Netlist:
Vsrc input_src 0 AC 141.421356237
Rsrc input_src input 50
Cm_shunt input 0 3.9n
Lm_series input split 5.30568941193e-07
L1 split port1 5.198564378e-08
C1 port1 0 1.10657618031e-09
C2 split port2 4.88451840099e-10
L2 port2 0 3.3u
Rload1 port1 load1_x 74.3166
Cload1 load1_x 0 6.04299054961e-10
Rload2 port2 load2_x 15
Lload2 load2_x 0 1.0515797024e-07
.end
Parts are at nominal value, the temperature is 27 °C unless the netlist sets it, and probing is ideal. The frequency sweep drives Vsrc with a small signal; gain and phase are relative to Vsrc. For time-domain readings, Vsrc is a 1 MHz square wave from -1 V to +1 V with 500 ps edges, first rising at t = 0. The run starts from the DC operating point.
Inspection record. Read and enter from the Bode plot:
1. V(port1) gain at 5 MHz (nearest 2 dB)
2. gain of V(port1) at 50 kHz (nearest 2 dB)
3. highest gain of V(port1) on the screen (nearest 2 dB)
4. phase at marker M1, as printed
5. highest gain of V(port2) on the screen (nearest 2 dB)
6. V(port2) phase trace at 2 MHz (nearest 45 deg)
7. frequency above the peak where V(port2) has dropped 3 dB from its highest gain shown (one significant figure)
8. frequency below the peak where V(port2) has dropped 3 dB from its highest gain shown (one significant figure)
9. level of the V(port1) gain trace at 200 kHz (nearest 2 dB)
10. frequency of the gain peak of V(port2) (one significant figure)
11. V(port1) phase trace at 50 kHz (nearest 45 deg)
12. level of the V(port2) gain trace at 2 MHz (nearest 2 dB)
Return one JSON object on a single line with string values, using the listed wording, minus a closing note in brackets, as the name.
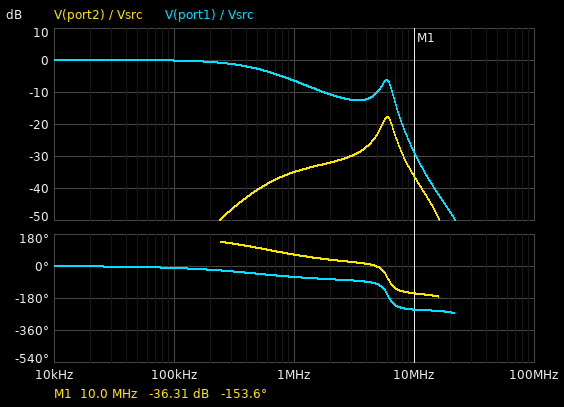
{"V(port1) gain at 5 MHz": "-10 dB", "gain of V(port1) at 50 kHz": "0 dB", "highest gain of V(port1) on the screen": "0 dB", "phase at marker M1, as printed": "-153.6 deg", "highest gain of V(port2) on the screen": "-18 dB", "V(port2) phase trace at 2 MHz": "45 deg", "frequency above the peak where V(port2) has dropped 3 dB from its highest gain shown": "7 MHz", "frequency below the peak where V(port2) has dropped 3 dB from its highest gain shown": "5 MHz", "level of the V(port1) gain trace at 200 kHz": "0 dB", "frequency of the gain peak of V(port2)": "6 MHz", "V(port1) phase trace at 50 kHz": "0 deg", "level of the V(port2) gain trace at 2 MHz": "-32 dB"}
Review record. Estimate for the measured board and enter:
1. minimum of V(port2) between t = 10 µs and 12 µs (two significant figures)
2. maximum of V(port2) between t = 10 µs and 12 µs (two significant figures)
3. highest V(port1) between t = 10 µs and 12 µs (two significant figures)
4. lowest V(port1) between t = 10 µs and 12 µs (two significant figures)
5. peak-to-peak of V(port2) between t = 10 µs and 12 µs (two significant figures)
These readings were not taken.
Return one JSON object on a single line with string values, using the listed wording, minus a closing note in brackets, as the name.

{"minimum of V(port2) between t = 10 µs and 12 µs": "-65 mV", "maximum of V(port2) between t = 10 µs and 12 µs": "65 mV", "highest V(port1) between t = 10 µs and 12 µs": "670 mV", "lowest V(port1) between t = 10 µs and 12 µs": "-670 mV", "peak-to-peak of V(port2) between t = 10 µs and 12 µs": "130 mV"}
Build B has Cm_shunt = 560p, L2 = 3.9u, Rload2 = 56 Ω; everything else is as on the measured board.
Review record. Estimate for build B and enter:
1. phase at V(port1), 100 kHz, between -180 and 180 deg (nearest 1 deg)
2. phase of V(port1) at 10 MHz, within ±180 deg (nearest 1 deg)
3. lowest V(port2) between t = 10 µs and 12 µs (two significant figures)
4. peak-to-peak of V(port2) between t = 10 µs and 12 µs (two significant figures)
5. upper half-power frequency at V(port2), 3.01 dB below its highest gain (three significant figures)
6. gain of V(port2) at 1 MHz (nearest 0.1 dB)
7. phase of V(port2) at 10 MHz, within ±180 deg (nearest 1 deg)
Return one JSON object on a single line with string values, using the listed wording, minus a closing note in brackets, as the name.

{"phase at V(port1), 100 kHz, between -180 and 180 deg": "-5 deg", "phase of V(port1) at 10 MHz, within ±180 deg": "-144 deg", "lowest V(port2) between t = 10 µs and 12 µs": "-330 mV", "peak-to-peak of V(port2) between t = 10 µs and 12 µs": "660 mV", "upper half-power frequency at V(port2), 3.01 dB below its highest gain": "11.4 MHz", "gain of V(port2) at 1 MHz": "-25.2 dB", "phase of V(port2) at 10 MHz, within ±180 deg": "-106 deg"}
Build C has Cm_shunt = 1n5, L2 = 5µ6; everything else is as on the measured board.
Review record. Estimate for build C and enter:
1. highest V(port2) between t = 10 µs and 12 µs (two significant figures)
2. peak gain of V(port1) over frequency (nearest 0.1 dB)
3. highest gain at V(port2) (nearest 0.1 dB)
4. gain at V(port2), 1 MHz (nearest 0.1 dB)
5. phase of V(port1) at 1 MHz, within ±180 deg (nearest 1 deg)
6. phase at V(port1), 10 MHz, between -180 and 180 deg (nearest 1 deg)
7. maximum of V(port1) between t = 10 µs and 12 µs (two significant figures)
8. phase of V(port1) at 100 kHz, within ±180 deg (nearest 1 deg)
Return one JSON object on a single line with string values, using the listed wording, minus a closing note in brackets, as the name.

{"highest V(port2) between t = 10 µs and 12 µs": "120 mV", "peak gain of V(port1) over frequency": "0 dB", "highest gain at V(port2)": "-15.3 dB", "gain at V(port2), 1 MHz": "-31.1 dB", "phase of V(port1) at 1 MHz, within ±180 deg": "-48 deg", "phase at V(port1), 10 MHz, between -180 and 180 deg": "131 deg", "maximum of V(port1) between t = 10 µs and 12 µs": "890 mV", "phase of V(port1) at 100 kHz, within ±180 deg": "-7 deg"}
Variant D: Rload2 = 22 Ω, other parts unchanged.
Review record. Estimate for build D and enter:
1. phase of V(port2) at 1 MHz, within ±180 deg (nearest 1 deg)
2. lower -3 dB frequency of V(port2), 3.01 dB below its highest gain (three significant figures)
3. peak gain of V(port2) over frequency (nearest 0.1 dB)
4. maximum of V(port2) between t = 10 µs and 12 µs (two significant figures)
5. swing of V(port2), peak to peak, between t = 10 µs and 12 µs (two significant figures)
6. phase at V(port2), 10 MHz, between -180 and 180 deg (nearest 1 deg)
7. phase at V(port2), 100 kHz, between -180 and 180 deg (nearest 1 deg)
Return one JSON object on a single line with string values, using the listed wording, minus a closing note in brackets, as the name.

{"phase of V(port2) at 1 MHz, within ±180 deg": "74 deg", "lower -3 dB frequency of V(port2), 3.01 dB below its highest gain": "5.24 MHz", "peak gain of V(port2) over frequency": "-15.6 dB", "maximum of V(port2) between t = 10 µs and 12 µs": "88 mV", "swing of V(port2), peak to peak, between t = 10 µs and 12 µs": "180 mV", "phase at V(port2), 10 MHz, between -180 and 180 deg": "-167 deg", "phase at V(port2), 100 kHz, between -180 and 180 deg": "164 deg"}
